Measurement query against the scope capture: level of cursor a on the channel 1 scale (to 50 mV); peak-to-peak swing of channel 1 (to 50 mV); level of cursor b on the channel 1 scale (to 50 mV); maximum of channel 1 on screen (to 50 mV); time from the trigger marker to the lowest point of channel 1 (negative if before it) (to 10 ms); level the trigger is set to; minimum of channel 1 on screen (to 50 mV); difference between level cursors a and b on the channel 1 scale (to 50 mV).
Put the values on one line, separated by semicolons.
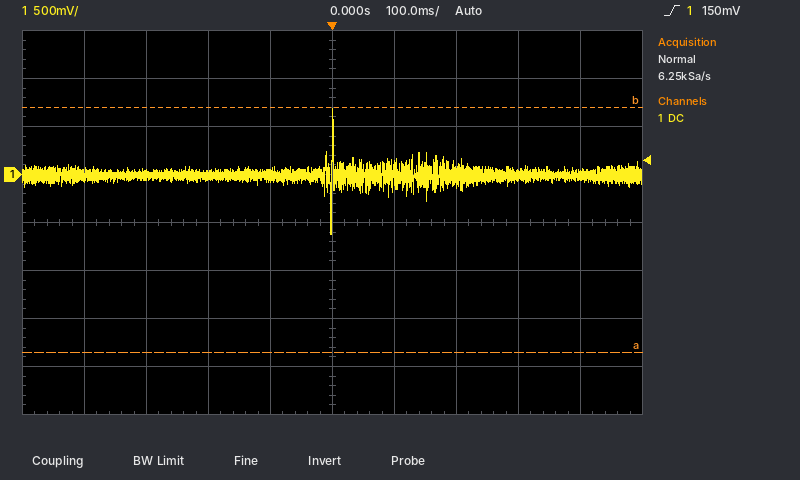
-1.85 V; 1.30 V; 700 mV; 700 mV; 0 ms; 150 mV; -600 mV; 2.55 V
